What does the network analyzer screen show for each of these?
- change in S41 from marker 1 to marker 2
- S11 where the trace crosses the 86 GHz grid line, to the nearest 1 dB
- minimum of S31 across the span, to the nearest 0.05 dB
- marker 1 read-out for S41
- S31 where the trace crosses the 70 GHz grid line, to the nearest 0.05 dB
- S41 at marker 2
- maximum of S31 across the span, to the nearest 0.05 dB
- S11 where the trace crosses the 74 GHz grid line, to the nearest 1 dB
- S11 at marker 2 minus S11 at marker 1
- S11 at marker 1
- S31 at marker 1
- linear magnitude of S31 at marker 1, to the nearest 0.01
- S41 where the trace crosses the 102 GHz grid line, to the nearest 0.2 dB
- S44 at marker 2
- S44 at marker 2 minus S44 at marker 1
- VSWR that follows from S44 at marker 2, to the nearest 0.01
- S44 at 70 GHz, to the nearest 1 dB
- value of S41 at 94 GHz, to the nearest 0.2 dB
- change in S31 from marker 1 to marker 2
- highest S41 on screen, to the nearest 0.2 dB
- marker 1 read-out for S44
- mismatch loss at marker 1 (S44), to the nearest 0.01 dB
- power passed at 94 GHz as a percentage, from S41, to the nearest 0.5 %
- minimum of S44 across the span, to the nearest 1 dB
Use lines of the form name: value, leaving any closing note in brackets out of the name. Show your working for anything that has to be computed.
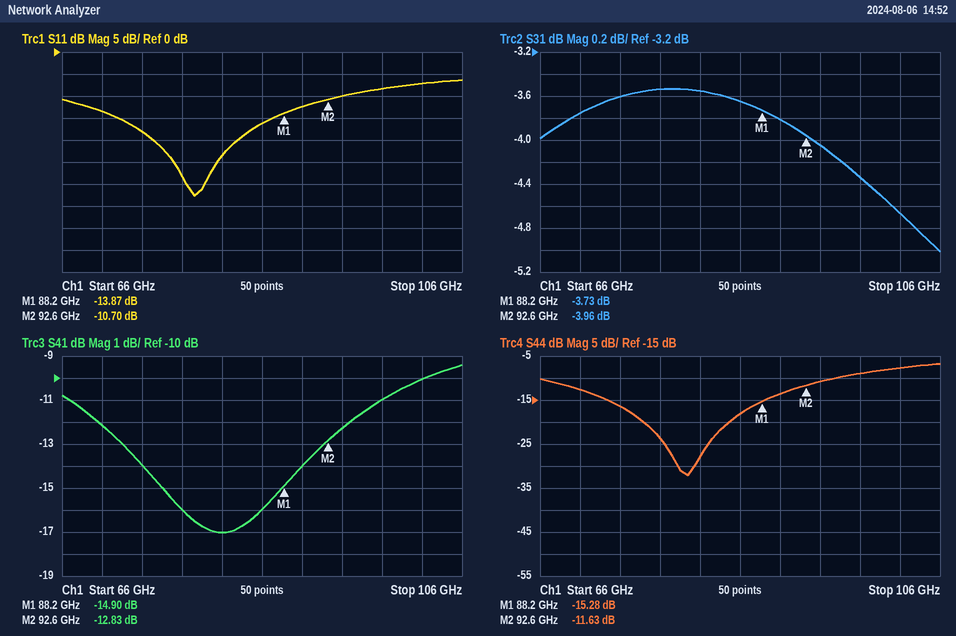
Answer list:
change in S41 from marker 1 to marker 2: -12.83 − (-14.9) = 2.07 dB
S11 where the trace crosses the 86 GHz grid line, to the nearest 1 dB: -16 dB
minimum of S31 across the span, to the nearest 0.05 dB: -5.00 dB
marker 1 read-out for S41: -14.90 dB
S31 where the trace crosses the 70 GHz grid line, to the nearest 0.05 dB: -3.75 dB
S41 at marker 2: -12.83 dB
maximum of S31 across the span, to the nearest 0.05 dB: -3.55 dB
S11 where the trace crosses the 74 GHz grid line, to the nearest 1 dB: -18 dB
S11 at marker 2 minus S11 at marker 1: -10.7 − (-13.87) = 3.17 dB
S11 at marker 1: -13.87 dB
S31 at marker 1: -3.73 dB
linear magnitude of S31 at marker 1, to the nearest 0.01: 10^(-3.73/20) ≈ 0.65
S41 where the trace crosses the 102 GHz grid line, to the nearest 0.2 dB: -10.0 dB
S44 at marker 2: -11.63 dB
S44 at marker 2 minus S44 at marker 1: -11.63 − (-15.28) = 3.65 dB
VSWR that follows from S44 at marker 2, to the nearest 0.01: (1 + 0.2621)/(1 − 0.2621) ≈ 1.71
S44 at 70 GHz, to the nearest 1 dB: -13 dB
value of S41 at 94 GHz, to the nearest 0.2 dB: -12.2 dB
change in S31 from marker 1 to marker 2: -3.96 − (-3.73) = -0.23 dB
highest S41 on screen, to the nearest 0.2 dB: -9.4 dB
marker 1 read-out for S44: -15.28 dB
mismatch loss at marker 1 (S44), to the nearest 0.01 dB: −10 log10(1 − 10^(-15.28/10)) ≈ 0.13 dB
power passed at 94 GHz as a percentage, from S41, to the nearest 0.5 %: 10^(-12.2/10) ≈ 6.0 %
minimum of S44 across the span, to the nearest 1 dB: -32 dB
